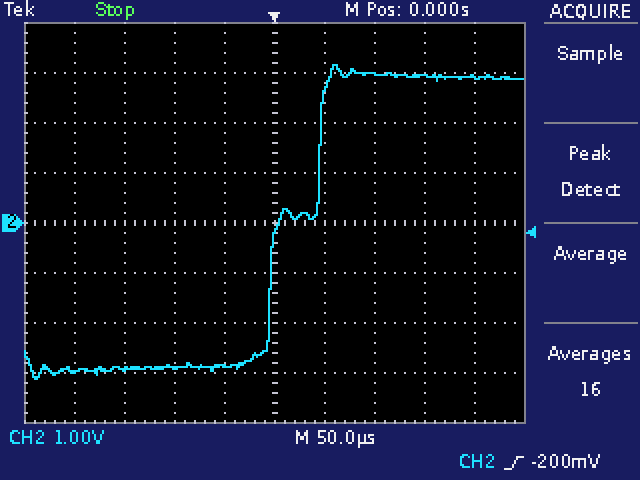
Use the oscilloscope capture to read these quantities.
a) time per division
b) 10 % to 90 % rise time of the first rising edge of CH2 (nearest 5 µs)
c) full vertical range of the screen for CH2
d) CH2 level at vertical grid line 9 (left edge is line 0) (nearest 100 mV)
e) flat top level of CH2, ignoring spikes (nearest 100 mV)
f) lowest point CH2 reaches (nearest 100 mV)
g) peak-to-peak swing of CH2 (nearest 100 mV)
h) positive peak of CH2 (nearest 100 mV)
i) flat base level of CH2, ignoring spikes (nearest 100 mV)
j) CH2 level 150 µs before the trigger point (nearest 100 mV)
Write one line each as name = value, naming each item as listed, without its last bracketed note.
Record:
time per division = 50 µs
10 % to 90 % rise time of the first rising edge of CH2 = 55 µs
full vertical range of the screen for CH2 = 8 V
CH2 level at vertical grid line 9 (left edge is line 0) = 2.9 V
flat top level of CH2, ignoring spikes = 2.9 V
lowest point CH2 reaches = -3.1 V
peak-to-peak swing of CH2 = 6.3 V
positive peak of CH2 = 3.2 V
flat base level of CH2, ignoring spikes = -2.9 V
CH2 level 150 µs before the trigger point = -2.9 V
